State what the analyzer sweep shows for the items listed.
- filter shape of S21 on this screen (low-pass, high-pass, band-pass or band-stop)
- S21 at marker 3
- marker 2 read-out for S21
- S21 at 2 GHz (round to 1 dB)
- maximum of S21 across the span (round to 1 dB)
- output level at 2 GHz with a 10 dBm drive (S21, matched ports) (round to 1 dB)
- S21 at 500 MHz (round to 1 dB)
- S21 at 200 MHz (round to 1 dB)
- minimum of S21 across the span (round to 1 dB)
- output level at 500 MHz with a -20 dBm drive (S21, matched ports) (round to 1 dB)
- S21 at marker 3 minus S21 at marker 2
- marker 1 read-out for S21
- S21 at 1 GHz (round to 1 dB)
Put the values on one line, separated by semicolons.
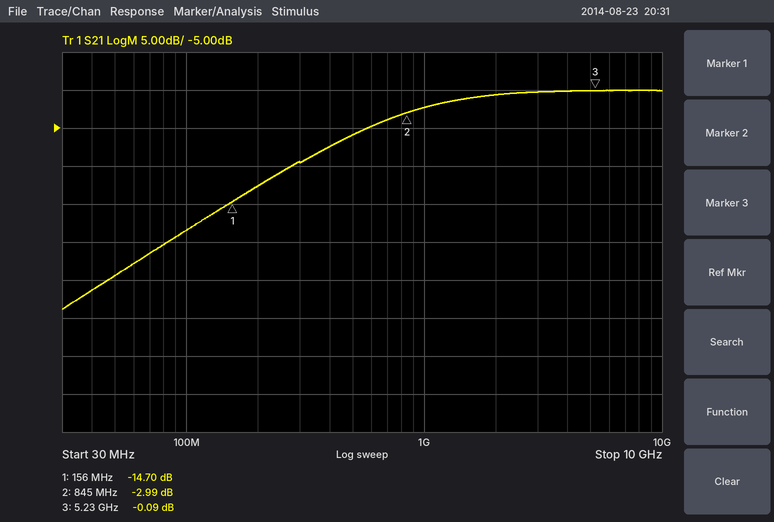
high-pass; -0.09 dB; -2.99 dB; -1 dB; 0 dB; 9 dBm; -6 dB; -13 dB; -29 dB; -26 dBm; 2.90 dB; -14.70 dB; -2 dB
